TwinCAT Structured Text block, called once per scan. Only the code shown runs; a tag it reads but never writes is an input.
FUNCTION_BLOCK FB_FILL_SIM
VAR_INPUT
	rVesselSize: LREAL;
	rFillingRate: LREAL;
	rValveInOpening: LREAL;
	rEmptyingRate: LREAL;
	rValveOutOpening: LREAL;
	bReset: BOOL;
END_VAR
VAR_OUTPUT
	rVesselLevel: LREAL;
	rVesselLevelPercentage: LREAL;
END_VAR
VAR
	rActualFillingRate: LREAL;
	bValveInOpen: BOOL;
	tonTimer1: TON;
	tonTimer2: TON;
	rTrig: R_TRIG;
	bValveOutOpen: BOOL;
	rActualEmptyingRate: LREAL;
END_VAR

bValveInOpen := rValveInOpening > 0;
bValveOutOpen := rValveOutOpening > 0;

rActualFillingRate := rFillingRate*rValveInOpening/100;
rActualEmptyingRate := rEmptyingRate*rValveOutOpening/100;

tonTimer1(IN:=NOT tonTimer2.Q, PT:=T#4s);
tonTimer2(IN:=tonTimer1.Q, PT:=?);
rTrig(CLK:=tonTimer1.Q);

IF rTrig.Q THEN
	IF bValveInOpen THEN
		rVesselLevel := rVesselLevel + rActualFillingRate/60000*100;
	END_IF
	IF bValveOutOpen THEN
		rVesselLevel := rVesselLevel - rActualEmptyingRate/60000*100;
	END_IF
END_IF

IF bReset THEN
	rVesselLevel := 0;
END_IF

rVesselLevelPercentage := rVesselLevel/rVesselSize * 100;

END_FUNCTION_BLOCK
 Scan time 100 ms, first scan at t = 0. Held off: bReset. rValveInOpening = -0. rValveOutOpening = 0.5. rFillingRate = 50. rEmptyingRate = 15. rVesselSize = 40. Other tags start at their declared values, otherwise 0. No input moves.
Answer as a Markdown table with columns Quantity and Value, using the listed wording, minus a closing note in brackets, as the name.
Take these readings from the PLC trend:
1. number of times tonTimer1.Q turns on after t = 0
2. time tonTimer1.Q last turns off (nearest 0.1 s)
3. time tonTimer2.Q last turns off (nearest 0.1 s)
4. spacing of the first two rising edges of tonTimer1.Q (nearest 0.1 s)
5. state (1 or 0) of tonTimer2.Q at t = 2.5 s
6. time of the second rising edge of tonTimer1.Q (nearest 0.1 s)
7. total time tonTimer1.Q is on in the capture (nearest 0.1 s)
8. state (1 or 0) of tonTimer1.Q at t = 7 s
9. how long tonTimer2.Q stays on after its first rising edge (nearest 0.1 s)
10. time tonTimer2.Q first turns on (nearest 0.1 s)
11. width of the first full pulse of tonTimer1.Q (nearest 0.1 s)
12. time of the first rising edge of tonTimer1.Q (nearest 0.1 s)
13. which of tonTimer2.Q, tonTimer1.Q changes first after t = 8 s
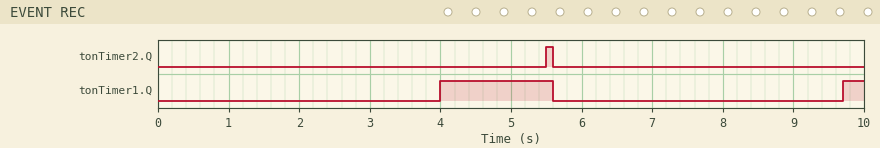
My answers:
| Quantity | Value |
|---|---|
| number of times tonTimer1.Q turns on after t = 0 | 2 |
| time tonTimer1.Q last turns off | 5.6 s |
| time tonTimer2.Q last turns off | 5.6 s |
| spacing of the first two rising edges of tonTimer1.Q | 5.7 s |
| state (1 or 0) of tonTimer2.Q at t = 2.5 s | 0 |
| time of the second rising edge of tonTimer1.Q | 9.7 s |
| total time tonTimer1.Q is on in the capture | 1.9 s |
| state (1 or 0) of tonTimer1.Q at t = 7 s | 0 |
| how long tonTimer2.Q stays on after its first rising edge | 0.1 s |
| time tonTimer2.Q first turns on | 5.5 s |
| width of the first full pulse of tonTimer1.Q | 1.6 s |
| time of the first rising edge of tonTimer1.Q | 4.0 s |
| which of tonTimer2.Q, tonTimer1.Q changes first after t = 8 s | tonTimer1.Q |
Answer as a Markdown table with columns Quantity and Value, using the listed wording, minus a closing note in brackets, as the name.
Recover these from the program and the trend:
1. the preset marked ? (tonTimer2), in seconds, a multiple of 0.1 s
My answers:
| Quantity | Value |
|---|---|
| the preset marked ? (tonTimer2), in seconds, a multiple of 0.1 s | 1.5 s |
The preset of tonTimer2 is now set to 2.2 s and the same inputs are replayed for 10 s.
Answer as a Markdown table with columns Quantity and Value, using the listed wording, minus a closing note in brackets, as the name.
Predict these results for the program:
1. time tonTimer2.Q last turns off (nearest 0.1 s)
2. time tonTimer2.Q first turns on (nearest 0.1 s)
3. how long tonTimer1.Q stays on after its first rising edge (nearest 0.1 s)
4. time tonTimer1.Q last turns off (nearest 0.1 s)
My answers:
| Quantity | Value |
|---|---|
| time tonTimer2.Q last turns off | 6.3 s |
| time tonTimer2.Q first turns on | 6.2 s |
| how long tonTimer1.Q stays on after its first rising edge | 2.3 s |
| time tonTimer1.Q last turns off | 6.3 s |
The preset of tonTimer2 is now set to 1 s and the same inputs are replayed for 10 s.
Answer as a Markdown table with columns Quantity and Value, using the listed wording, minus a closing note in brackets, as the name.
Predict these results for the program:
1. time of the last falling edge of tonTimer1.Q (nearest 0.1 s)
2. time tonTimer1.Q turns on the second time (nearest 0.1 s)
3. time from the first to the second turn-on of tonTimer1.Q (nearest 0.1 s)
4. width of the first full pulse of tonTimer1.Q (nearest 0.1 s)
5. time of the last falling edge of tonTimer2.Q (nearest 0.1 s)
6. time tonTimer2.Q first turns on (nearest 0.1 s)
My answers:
| Quantity | Value |
|---|---|
| time of the last falling edge of tonTimer1.Q | 5.1 s |
| time tonTimer1.Q turns on the second time | 9.2 s |
| time from the first to the second turn-on of tonTimer1.Q | 5.2 s |
| width of the first full pulse of tonTimer1.Q | 1.1 s |
| time of the last falling edge of tonTimer2.Q | 5.1 s |
| time tonTimer2.Q first turns on | 5.0 s |
